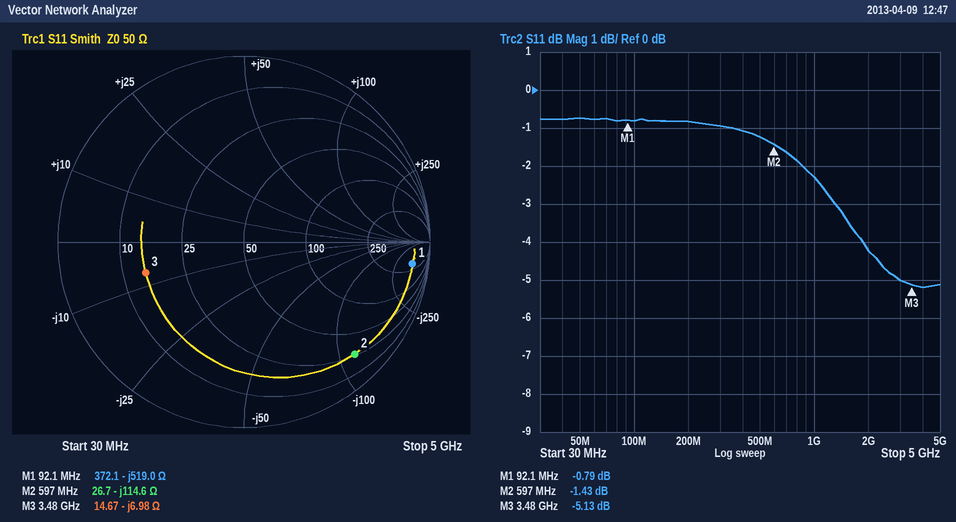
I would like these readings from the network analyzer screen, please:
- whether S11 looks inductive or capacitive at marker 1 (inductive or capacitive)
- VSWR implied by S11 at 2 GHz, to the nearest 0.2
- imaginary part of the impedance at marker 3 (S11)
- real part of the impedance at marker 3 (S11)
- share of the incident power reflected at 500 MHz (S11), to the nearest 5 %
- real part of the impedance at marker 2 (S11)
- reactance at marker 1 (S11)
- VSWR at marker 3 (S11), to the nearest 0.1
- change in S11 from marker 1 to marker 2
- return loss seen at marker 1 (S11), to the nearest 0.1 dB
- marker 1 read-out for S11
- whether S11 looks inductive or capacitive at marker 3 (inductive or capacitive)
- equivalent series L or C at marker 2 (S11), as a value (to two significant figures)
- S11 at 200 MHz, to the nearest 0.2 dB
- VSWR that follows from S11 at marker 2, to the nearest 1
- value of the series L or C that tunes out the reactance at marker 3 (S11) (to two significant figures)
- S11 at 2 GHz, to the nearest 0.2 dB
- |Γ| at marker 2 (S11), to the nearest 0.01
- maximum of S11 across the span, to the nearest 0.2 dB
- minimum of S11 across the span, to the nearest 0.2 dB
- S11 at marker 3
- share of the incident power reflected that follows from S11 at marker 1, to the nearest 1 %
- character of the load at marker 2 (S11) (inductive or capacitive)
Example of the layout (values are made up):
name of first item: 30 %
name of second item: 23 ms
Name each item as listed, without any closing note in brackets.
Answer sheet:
whether S11 looks inductive or capacitive at marker 1: capacitive
VSWR implied by S11 at 2 GHz, to the nearest 0.2: 4.2
imaginary part of the impedance at marker 3: -6.98 Ω
real part of the impedance at marker 3: 14.67 Ω
share of the incident power reflected at 500 MHz (S11), to the nearest 5 %: 75 %
real part of the impedance at marker 2: 26.7 Ω
reactance at marker 1: -519.0 Ω
VSWR at marker 3 (S11), to the nearest 0.1: 3.5
change in S11 from marker 1 to marker 2: -0.64 dB
return loss seen at marker 1 (S11), to the nearest 0.1 dB: 0.8 dB
marker 1 read-out for S11: -0.79 dB
whether S11 looks inductive or capacitive at marker 3: capacitive
equivalent series L or C at marker 2 (S11), as a value: 2.3 pF
S11 at 200 MHz, to the nearest 0.2 dB: -0.8 dB
VSWR that follows from S11 at marker 2, to the nearest 1: 12
value of the series L or C that tunes out the reactance at marker 3 (S11): 320 pH
S11 at 2 GHz, to the nearest 0.2 dB: -4.2 dB
|Γ| at marker 2 (S11), to the nearest 0.01: 0.85
maximum of S11 across the span, to the nearest 0.2 dB: -0.8 dB
minimum of S11 across the span, to the nearest 0.2 dB: -5.2 dB
S11 at marker 3: -5.13 dB
share of the incident power reflected that follows from S11 at marker 1, to the nearest 1 %: 83 %
character of the load at marker 2 (S11): capacitive
